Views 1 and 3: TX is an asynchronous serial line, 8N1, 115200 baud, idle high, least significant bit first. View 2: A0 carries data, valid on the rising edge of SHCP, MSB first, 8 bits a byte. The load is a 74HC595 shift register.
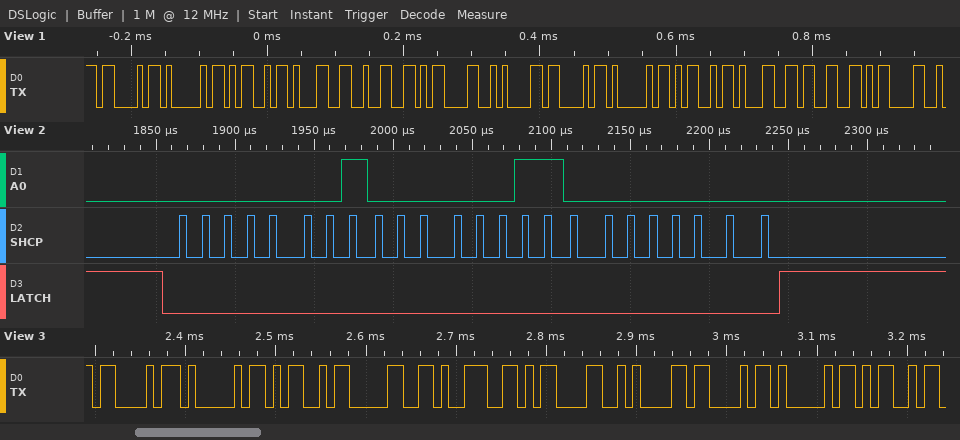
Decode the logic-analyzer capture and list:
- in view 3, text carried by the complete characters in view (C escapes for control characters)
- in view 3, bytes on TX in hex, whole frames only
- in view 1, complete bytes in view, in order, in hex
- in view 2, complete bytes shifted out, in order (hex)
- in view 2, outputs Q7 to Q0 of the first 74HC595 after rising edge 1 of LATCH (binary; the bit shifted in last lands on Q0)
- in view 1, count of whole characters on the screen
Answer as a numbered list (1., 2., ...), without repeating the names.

1. "CAM09\r\nCAM"
2. 0x43 0x41 0x4D 0x30 0x39 0x0D 0x0A 0x43 0x41 0x4D
3. 43 41 4D 31 32 0D 0A 43 41 4D 31 33 0D
4. 01 03 00
5. 00000000
6. 13
